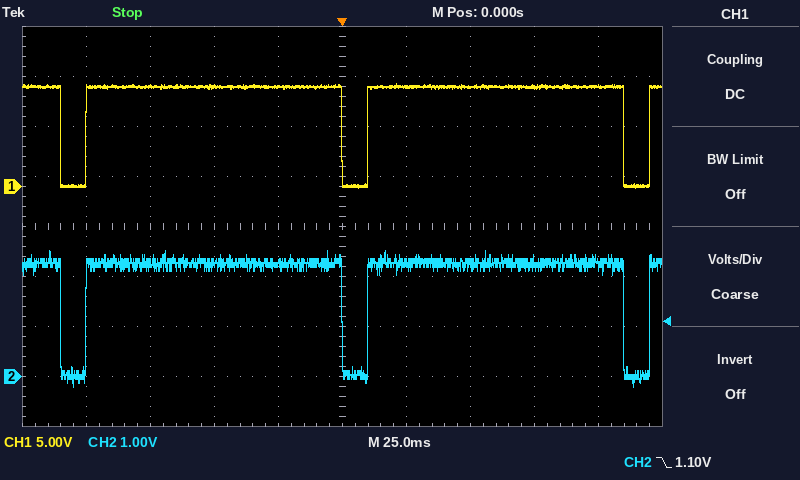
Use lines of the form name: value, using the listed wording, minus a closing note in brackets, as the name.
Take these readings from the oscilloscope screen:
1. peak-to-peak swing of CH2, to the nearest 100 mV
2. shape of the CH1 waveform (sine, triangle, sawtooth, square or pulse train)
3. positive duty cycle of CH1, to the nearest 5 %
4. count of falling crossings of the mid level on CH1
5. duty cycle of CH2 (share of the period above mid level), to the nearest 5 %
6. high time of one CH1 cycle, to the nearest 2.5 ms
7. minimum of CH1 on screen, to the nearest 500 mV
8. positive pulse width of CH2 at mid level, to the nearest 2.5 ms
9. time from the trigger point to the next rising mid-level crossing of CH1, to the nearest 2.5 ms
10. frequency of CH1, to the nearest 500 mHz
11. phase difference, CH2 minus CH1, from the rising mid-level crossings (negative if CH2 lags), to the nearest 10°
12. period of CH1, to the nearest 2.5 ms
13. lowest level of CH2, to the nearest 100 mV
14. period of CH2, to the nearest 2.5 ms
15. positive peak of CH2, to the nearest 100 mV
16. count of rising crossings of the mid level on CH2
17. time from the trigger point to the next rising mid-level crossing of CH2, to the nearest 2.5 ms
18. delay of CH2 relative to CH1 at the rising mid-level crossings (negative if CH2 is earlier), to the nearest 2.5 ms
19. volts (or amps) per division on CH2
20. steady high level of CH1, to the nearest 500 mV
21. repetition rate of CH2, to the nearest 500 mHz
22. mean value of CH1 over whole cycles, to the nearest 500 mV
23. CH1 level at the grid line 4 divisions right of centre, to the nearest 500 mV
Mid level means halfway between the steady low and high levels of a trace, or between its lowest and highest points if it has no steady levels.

peak-to-peak swing of CH2, to the nearest 100 mV: 2.7 V
shape of the CH1 waveform: pulse train
positive duty cycle of CH1, to the nearest 5 %: 90 %
count of falling crossings of the mid level on CH1: 3
duty cycle of CH2 (share of the period above mid level), to the nearest 5 %: 90 %
high time of one CH1 cycle, to the nearest 2.5 ms: 100.0 ms
minimum of CH1 on screen, to the nearest 500 mV: 0.0 V
positive pulse width of CH2 at mid level, to the nearest 2.5 ms: 100.0 ms
time from the trigger point to the next rising mid-level crossing of CH1, to the nearest 2.5 ms: 10.0 ms
frequency of CH1, to the nearest 500 mHz: 9.0 Hz
phase difference, CH2 minus CH1, from the rising mid-level crossings (negative if CH2 lags), to the nearest 10°: 0°
period of CH1, to the nearest 2.5 ms: 110.0 ms
lowest level of CH2, to the nearest 100 mV: -200 mV
period of CH2, to the nearest 2.5 ms: 110.0 ms
positive peak of CH2, to the nearest 100 mV: 2.5 V
count of rising crossings of the mid level on CH2: 3
time from the trigger point to the next rising mid-level crossing of CH2, to the nearest 2.5 ms: 10.0 ms
delay of CH2 relative to CH1 at the rising mid-level crossings (negative if CH2 is earlier), to the nearest 2.5 ms: 0.0 ms
volts (or amps) per division on CH2: 1 V
steady high level of CH1, to the nearest 500 mV: 10.0 V
repetition rate of CH2, to the nearest 500 mHz: 9.0 Hz
mean value of CH1 over whole cycles, to the nearest 500 mV: 9.0 V
CH1 level at the grid line 4 divisions right of centre, to the nearest 500 mV: 10.0 V
